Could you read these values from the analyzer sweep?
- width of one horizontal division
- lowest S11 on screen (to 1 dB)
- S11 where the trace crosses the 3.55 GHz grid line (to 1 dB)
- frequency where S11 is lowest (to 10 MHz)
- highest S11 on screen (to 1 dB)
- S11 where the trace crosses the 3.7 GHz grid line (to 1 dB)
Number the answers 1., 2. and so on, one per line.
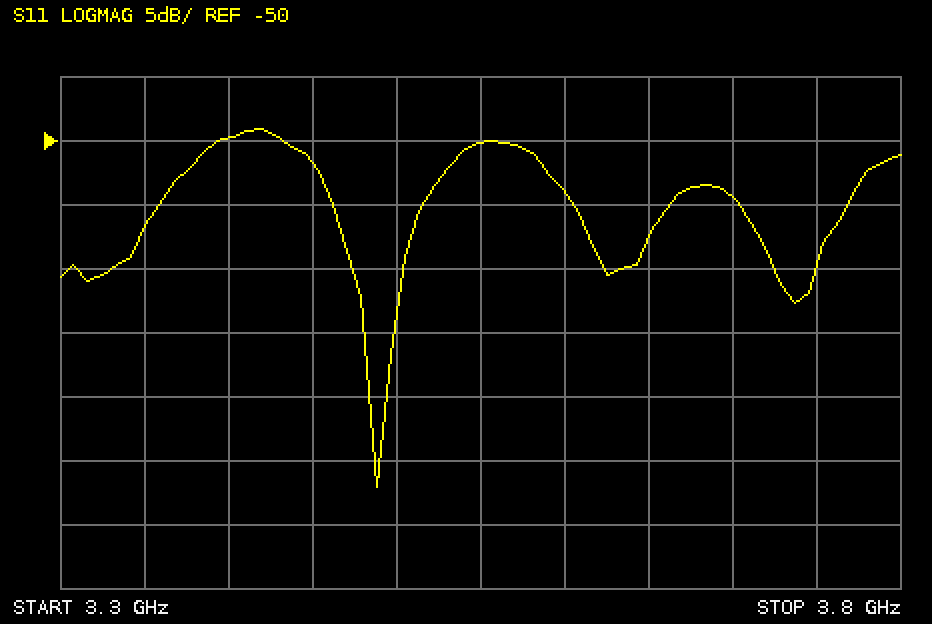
1. 50 MHz
2. -77 dB
3. -50 dB
4. 3.49 GHz
5. -49 dB
6. -54 dB
